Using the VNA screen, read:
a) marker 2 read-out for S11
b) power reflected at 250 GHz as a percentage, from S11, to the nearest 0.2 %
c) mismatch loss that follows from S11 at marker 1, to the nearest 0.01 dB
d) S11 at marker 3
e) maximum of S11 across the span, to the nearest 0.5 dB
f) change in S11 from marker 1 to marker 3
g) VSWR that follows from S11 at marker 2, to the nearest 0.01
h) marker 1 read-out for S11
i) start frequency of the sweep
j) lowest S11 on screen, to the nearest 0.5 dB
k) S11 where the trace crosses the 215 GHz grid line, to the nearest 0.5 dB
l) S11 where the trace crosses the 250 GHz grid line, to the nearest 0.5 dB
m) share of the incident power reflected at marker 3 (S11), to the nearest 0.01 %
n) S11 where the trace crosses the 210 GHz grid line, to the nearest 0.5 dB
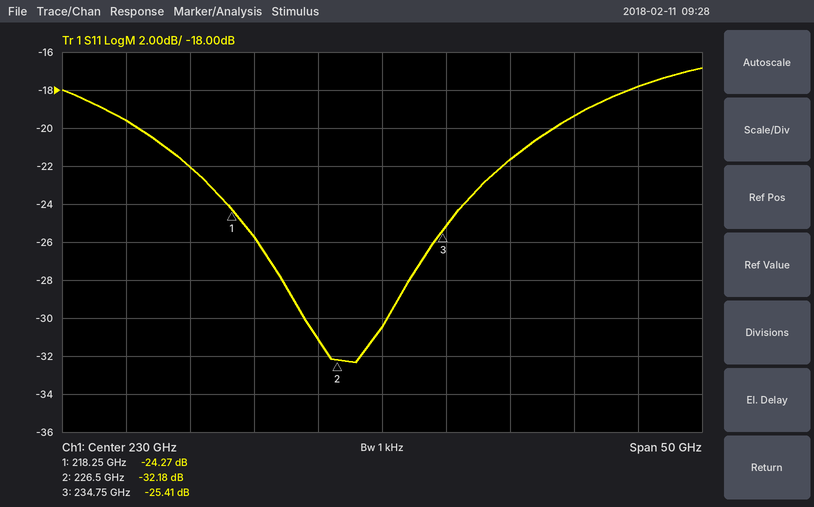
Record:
-32.18 dB
1.6 %
0.02 dB
-25.41 dB
-17.0 dB
-1.14 dB
1.05
-24.27 dB
205 GHz
-32.5 dB
-22.0 dB
-18.0 dB
0.29 %
-19.5 dB
